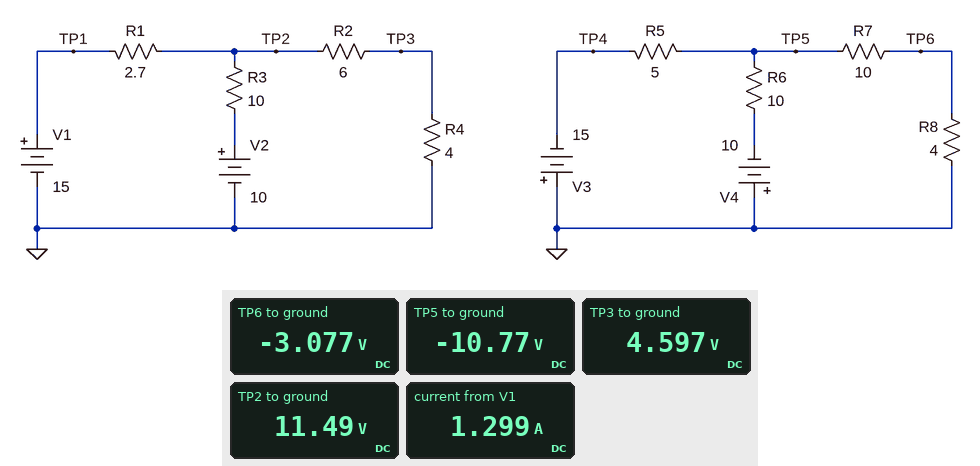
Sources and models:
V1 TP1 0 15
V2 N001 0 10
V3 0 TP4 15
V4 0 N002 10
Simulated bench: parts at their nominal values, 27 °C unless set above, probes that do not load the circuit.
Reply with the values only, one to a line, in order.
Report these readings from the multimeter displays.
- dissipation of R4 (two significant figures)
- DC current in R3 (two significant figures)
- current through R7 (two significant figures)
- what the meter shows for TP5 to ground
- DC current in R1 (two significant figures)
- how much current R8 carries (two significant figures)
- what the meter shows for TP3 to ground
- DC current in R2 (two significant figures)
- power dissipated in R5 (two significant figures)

5.3 W
150 mA
770 mA
-10.77 V
1.3 A
770 mA
4.597 V
1.1 A
3.6 W
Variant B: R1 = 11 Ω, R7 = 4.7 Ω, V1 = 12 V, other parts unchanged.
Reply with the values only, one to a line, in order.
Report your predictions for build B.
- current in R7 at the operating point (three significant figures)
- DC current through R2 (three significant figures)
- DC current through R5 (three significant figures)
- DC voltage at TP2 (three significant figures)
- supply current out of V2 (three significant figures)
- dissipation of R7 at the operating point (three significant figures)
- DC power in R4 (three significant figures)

1.11 A
719 mA
1.07 A
7.19 V
281 mA
5.77 W
2.07 W
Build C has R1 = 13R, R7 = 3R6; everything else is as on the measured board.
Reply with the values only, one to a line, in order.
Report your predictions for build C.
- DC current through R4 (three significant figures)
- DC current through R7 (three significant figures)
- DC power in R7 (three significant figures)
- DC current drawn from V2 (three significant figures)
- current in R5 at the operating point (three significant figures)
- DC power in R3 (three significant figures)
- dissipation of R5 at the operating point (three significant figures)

778 mA
1.22 A
5.35 W
222 mA
1.15 A
494 mW
6.57 W
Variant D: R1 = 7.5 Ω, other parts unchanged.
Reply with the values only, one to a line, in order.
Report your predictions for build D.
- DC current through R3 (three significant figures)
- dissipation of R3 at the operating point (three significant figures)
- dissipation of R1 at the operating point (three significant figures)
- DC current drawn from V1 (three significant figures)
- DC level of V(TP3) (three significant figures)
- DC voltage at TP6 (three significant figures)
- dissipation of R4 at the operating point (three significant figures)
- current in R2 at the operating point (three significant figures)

100 mA
100 mW
4.80 W
800 mA
3.60 V
-3.08 V
3.24 W
900 mA
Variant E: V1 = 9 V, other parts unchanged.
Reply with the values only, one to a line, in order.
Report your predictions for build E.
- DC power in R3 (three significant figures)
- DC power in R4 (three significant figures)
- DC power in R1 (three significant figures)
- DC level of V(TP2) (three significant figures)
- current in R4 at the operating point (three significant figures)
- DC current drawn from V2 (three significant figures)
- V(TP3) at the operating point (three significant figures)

577 mW
2.31 W
729 mW
7.60 V
760 mA
240 mA
3.04 V
